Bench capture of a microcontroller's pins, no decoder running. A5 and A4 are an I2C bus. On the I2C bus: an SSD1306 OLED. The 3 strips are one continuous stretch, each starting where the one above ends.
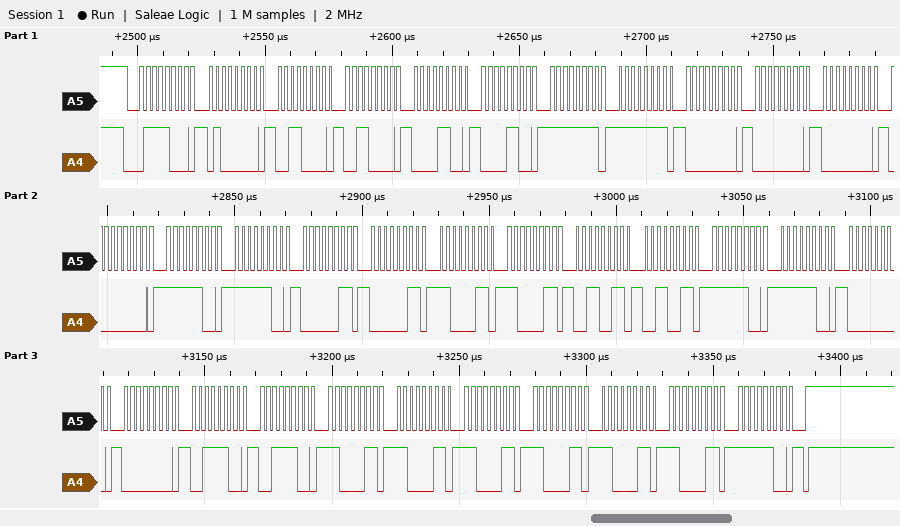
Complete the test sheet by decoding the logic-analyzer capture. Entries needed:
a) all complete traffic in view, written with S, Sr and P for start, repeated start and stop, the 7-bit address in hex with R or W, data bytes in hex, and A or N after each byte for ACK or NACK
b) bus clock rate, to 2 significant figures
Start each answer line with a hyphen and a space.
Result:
- S 3CW A 40 A 30 A 30 A 0C A 0C A FF A FF A 00 A 00 A 00 A 00 A FC A FC A 03 A 03 A C3 A C3 A 33 A 33 A FC A FC A 00 A 00 A 3C A 3C A C3 A C3 A C3 A C3 A C3 A C3 A FC A P
- 400 kHz
